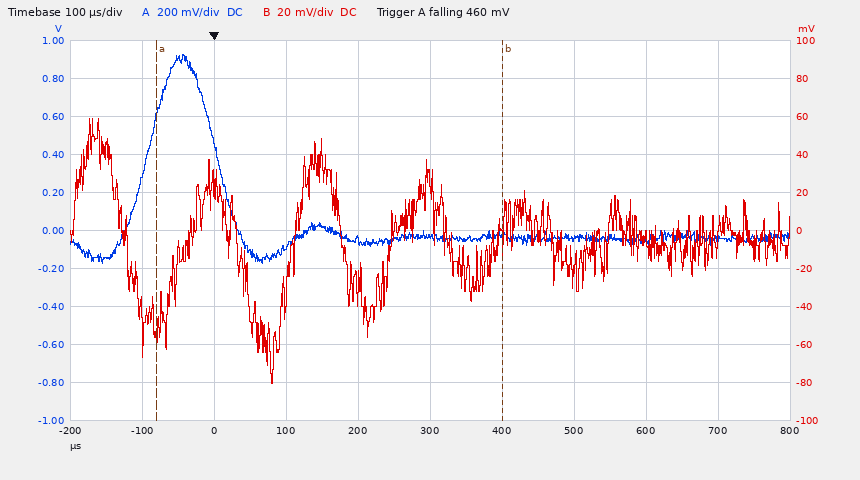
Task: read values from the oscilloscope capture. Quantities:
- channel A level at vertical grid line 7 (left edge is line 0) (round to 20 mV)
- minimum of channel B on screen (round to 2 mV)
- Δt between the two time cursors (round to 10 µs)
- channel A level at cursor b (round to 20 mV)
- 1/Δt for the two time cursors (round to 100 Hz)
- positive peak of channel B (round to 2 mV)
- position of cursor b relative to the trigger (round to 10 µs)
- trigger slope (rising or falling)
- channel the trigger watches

-40 mV
-80 mV
480 µs
-20 mV
2.1 kHz
58 mV
+400 µs
falling
channel A
